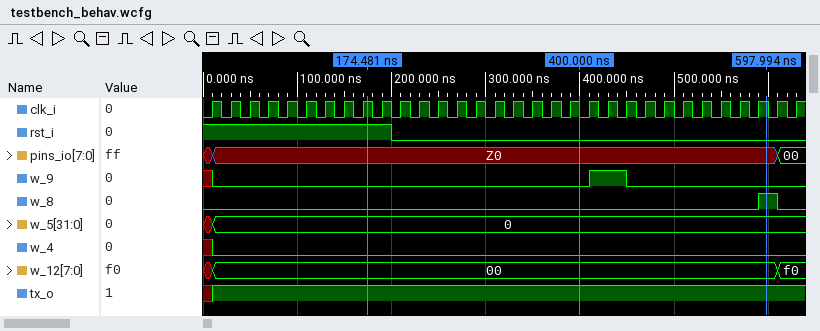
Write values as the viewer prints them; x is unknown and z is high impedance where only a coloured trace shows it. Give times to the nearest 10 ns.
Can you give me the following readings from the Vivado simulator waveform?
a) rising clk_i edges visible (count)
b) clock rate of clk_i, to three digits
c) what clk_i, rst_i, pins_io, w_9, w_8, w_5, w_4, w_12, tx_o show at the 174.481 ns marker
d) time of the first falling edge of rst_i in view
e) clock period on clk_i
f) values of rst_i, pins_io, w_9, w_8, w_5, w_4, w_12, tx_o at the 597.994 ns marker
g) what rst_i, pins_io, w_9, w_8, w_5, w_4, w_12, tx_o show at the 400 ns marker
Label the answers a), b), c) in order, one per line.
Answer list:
a) 32
b) 50.0 MHz
c) clk_i=1, rst_i=1, pins_io=Z0, w_9=0, w_8=0, w_5=0, w_4=0, w_12=00, tx_o=1
d) 200 ns
e) 20 ns
f) rst_i=0, pins_io=Z0, w_9=0, w_8=1, w_5=0, w_4=0, w_12=00, tx_o=1
g) rst_i=0, pins_io=Z0, w_9=0, w_8=0, w_5=0, w_4=0, w_12=00, tx_o=1
